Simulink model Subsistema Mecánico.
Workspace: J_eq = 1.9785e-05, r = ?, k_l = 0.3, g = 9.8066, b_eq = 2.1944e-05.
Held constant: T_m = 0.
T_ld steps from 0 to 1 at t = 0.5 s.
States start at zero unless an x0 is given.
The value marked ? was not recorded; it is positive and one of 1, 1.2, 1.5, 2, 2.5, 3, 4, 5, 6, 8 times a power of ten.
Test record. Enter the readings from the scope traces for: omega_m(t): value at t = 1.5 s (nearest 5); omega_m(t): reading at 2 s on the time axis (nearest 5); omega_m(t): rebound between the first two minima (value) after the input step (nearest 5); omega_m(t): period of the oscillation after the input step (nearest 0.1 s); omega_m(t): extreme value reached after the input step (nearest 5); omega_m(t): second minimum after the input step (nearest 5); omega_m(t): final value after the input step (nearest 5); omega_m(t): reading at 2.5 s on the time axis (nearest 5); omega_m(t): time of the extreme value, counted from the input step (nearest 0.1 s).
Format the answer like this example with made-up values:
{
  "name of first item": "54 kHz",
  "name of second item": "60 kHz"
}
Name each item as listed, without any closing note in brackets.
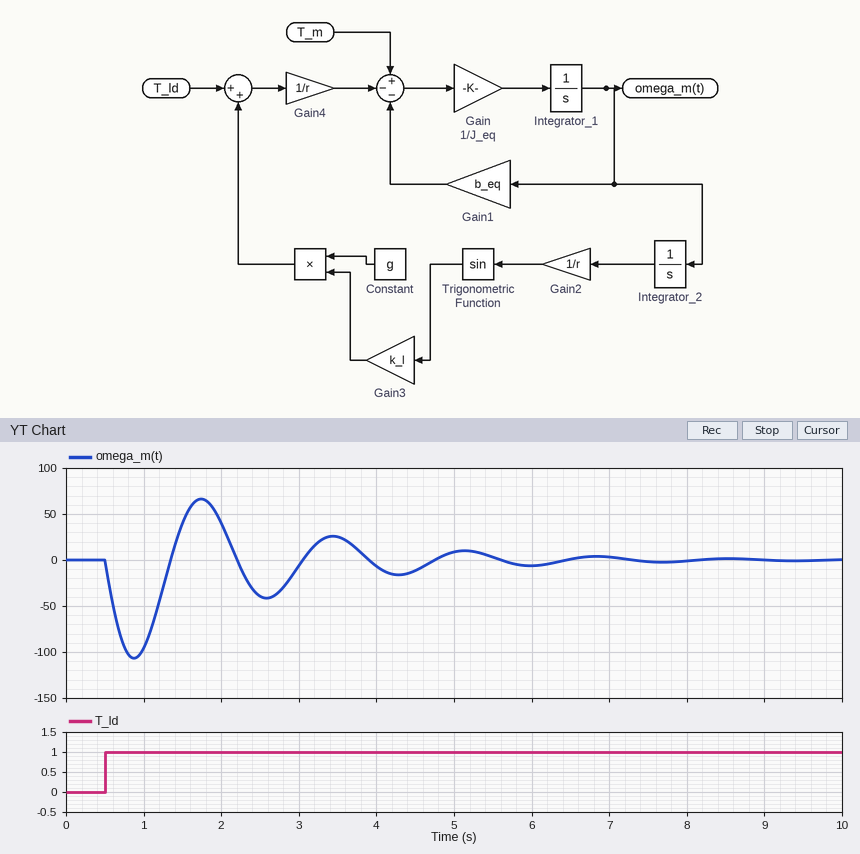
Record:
{
  "omega_m(t): value at t = 1.5 s": "40",
  "omega_m(t): reading at 2 s on the time axis": "40",
  "omega_m(t): rebound between the first two minima (value) after the input step": "65",
  "omega_m(t): period of the oscillation after the input step": "1.7 s",
  "omega_m(t): extreme value reached after the input step": "-105",
  "omega_m(t): second minimum after the input step": "-40",
  "omega_m(t): final value after the input step": "0",
  "omega_m(t): reading at 2.5 s on the time axis": "-40",
  "omega_m(t): time of the extreme value, counted from the input step": "0.4 s"
}
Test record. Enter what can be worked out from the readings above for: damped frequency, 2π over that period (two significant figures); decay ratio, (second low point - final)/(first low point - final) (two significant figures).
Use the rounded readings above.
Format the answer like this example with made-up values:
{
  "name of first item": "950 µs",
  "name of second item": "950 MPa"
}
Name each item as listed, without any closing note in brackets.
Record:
{
  "damped frequency, 2π over that period": "3.7 rad/s",
  "decay ratio, (second low point - final)/(first low point - final)": "0.38"
}
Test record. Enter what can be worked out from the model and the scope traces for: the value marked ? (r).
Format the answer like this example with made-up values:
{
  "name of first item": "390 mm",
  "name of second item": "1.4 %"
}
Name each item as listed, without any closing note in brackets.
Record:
{
  "the value marked ?": "100"
}
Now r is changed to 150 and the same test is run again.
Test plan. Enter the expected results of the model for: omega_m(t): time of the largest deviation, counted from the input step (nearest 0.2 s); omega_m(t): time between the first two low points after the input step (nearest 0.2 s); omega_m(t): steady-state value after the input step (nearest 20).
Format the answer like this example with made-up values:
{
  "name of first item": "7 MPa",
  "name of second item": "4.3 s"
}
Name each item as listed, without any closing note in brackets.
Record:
{
  "omega_m(t): time of the largest deviation, counted from the input step": "0.6 s",
  "omega_m(t): time between the first two low points after the input step": "2.6 s",
  "omega_m(t): steady-state value after the input step": "0"
}
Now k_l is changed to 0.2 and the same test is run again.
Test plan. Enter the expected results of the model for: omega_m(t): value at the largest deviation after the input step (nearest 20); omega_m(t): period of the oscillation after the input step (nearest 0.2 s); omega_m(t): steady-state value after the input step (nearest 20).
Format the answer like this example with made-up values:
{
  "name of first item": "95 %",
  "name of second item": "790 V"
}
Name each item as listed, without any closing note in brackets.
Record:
{
  "omega_m(t): value at the largest deviation after the input step": "-120",
  "omega_m(t): period of the oscillation after the input step": "2.2 s",
  "omega_m(t): steady-state value after the input step": "0"
}
